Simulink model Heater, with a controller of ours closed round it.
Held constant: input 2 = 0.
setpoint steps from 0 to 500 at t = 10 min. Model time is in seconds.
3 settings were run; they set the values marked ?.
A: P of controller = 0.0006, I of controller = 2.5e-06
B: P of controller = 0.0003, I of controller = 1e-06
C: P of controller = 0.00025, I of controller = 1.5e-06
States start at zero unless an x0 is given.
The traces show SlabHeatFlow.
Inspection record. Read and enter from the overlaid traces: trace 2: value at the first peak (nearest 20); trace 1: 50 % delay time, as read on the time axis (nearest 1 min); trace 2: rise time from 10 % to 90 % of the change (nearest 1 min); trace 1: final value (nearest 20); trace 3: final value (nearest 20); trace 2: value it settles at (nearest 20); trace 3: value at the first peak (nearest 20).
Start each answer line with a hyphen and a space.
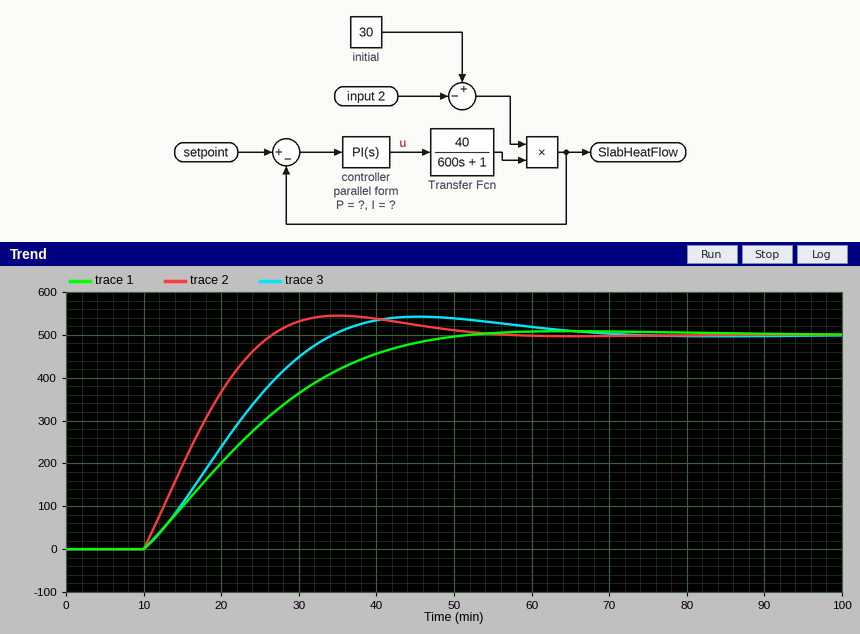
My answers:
- 540
- 23 min
- 12 min
- 500
- 500
- 500
- 540
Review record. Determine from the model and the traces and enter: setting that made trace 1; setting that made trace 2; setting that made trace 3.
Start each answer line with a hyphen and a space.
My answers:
- B
- A
- C
